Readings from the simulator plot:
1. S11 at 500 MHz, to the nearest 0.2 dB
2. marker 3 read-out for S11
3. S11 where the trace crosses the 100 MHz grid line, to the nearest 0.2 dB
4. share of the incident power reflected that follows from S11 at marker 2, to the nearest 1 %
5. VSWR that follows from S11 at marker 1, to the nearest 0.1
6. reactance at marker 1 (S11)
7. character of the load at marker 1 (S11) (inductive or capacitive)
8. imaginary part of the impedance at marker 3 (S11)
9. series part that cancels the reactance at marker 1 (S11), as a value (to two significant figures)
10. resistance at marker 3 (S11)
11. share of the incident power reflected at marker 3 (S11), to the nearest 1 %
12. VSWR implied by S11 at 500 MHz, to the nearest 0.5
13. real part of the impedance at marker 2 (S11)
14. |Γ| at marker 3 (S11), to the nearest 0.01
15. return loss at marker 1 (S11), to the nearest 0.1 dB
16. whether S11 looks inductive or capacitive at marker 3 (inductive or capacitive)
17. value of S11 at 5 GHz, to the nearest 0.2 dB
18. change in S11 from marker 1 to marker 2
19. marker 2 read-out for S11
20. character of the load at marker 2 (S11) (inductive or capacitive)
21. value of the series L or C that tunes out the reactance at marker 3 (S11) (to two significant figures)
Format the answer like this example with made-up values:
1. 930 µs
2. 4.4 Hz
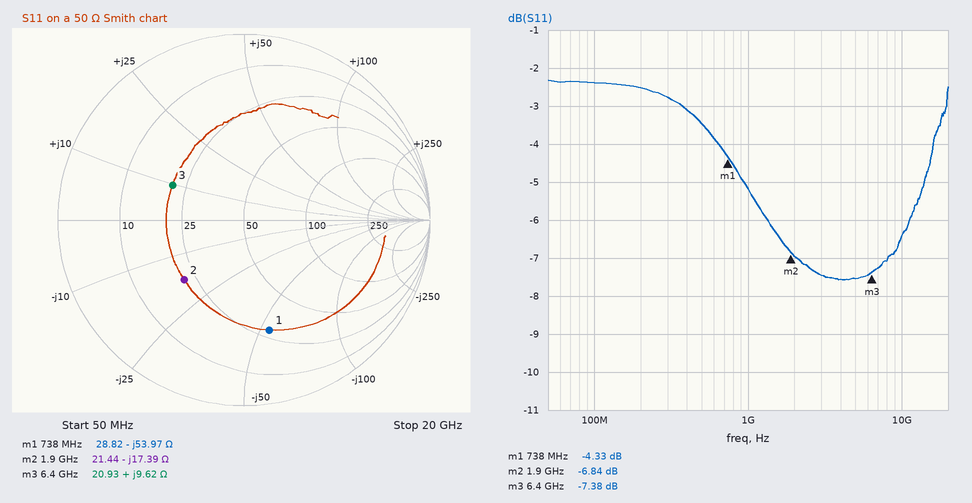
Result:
1. -3.4 dB
2. -7.38 dB
3. -2.4 dB
4. 21 %
5. 4.1
6. -53.97 Ω
7. capacitive
8. +9.62 Ω
9. 12 nH
10. 20.93 Ω
11. 18 %
12. 5.0
13. 21.44 Ω
14. 0.43
15. 4.3 dB
16. inductive
17. -7.6 dB
18. -2.51 dB
19. -6.84 dB
20. capacitive
21. 2.6 pF
